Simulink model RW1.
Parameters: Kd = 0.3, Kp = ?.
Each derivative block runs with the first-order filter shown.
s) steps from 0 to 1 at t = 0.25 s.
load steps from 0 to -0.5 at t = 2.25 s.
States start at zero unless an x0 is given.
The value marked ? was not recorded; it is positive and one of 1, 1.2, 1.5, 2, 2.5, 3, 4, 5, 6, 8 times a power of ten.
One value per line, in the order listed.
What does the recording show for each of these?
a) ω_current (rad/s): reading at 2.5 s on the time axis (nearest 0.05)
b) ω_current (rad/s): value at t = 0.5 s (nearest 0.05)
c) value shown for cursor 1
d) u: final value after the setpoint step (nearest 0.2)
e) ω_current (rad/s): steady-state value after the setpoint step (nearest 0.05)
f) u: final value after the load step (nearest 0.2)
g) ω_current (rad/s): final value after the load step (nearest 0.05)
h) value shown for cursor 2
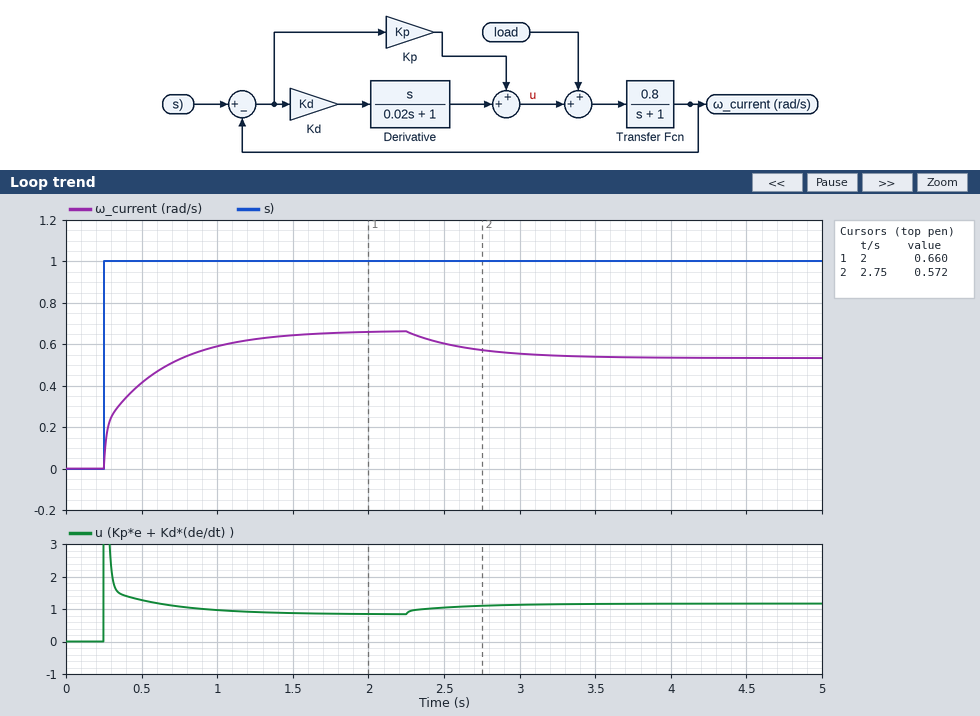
0.60
0.40
0.660
0.8
0.65
1.2
0.55
0.572
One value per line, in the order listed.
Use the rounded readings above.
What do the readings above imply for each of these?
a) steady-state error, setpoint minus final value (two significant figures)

0.35
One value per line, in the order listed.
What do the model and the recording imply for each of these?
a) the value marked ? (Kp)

2.5
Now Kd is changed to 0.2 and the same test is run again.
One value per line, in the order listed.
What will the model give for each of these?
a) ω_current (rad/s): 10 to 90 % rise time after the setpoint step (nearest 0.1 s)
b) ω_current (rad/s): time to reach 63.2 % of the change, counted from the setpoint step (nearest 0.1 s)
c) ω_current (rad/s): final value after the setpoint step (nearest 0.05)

0.8 s
0.3 s
0.65
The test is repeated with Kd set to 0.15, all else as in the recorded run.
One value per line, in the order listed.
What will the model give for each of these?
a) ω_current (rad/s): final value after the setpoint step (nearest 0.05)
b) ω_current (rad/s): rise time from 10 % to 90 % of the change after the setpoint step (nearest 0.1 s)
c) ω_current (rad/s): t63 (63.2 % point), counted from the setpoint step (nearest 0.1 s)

0.65
0.8 s
0.3 s
